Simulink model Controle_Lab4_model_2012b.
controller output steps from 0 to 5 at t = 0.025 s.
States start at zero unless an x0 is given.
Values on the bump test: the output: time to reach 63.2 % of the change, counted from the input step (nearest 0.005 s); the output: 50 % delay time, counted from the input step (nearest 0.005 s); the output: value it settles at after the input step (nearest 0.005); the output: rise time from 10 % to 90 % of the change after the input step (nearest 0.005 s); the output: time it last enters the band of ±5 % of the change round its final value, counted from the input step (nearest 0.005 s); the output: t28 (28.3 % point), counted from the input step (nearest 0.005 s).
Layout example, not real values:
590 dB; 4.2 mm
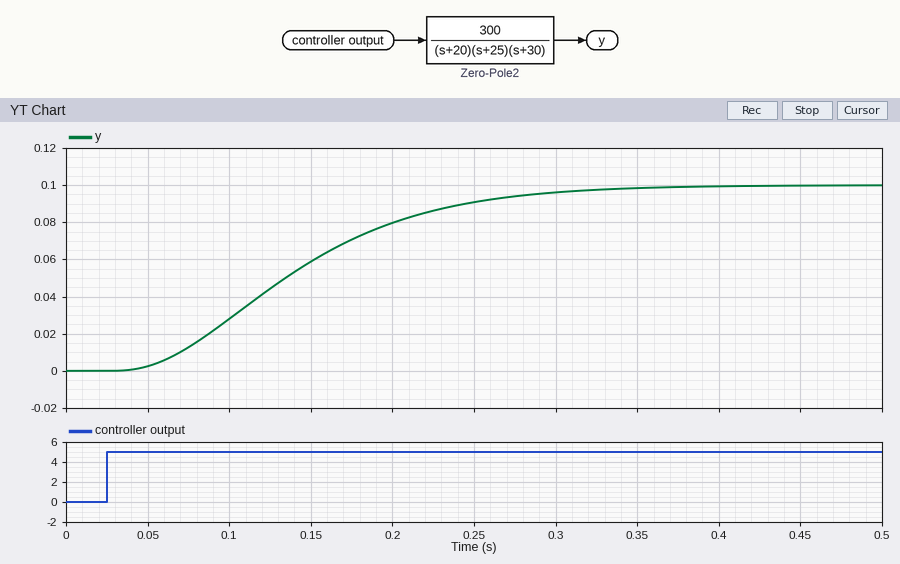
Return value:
0.135 s; 0.110 s; 0.100; 0.175 s; 0.260 s; 0.075 s
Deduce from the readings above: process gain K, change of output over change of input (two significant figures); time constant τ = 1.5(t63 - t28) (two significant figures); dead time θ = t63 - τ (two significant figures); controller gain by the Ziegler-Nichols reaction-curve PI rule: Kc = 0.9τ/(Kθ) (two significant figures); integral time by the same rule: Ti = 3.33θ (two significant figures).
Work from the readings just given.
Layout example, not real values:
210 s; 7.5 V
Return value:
0.020; 0.090 s; 0.045 s; 90; 0.15 s
